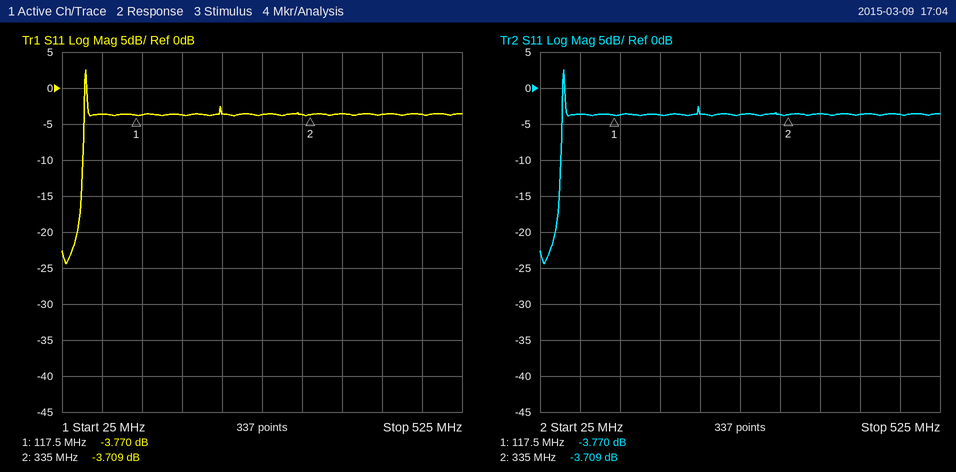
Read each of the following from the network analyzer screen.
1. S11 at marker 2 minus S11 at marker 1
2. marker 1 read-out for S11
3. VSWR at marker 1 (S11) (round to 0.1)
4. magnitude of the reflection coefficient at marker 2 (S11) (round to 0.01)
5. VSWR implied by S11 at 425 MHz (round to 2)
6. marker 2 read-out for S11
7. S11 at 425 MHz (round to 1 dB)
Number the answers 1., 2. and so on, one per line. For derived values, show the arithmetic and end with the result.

1. -3.709 − (-3.77) = 0.061 dB
2. -3.770 dB
3. (1 + 0.6479)/(1 − 0.6479) ≈ 4.7
4. 10^(-3.709/20) ≈ 0.65
5. |Γ| = 10^(-4/20) = 0.6310; VSWR = (1 + 0.6310)/(1 − 0.6310) ≈ 4
6. -3.709 dB
7. -4 dB
